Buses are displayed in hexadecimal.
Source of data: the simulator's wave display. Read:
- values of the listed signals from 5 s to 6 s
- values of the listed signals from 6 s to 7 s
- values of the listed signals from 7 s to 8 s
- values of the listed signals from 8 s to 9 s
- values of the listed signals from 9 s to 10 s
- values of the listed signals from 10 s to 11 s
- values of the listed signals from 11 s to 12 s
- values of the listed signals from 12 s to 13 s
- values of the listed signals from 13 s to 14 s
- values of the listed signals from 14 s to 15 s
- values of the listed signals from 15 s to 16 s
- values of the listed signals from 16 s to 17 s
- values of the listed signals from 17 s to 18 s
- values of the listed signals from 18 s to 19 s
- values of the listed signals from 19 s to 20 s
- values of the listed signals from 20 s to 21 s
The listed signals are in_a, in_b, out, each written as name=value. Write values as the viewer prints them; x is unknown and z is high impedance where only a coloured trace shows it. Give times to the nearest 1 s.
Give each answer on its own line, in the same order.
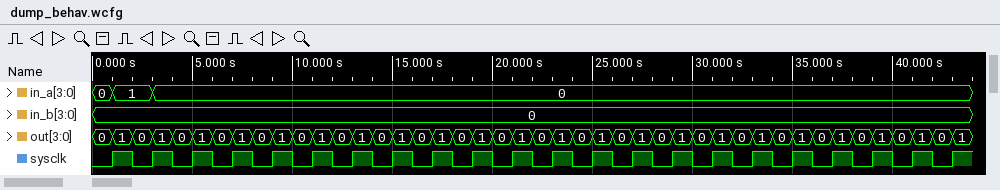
in_a=0, in_b=0, out=1
in_a=0, in_b=0, out=0
in_a=0, in_b=0, out=1
in_a=0, in_b=0, out=0
in_a=0, in_b=0, out=1
in_a=0, in_b=0, out=0
in_a=0, in_b=0, out=1
in_a=0, in_b=0, out=0
in_a=0, in_b=0, out=1
in_a=0, in_b=0, out=0
in_a=0, in_b=0, out=1
in_a=0, in_b=0, out=0
in_a=0, in_b=0, out=1
in_a=0, in_b=0, out=0
in_a=0, in_b=0, out=1
in_a=0, in_b=0, out=0
